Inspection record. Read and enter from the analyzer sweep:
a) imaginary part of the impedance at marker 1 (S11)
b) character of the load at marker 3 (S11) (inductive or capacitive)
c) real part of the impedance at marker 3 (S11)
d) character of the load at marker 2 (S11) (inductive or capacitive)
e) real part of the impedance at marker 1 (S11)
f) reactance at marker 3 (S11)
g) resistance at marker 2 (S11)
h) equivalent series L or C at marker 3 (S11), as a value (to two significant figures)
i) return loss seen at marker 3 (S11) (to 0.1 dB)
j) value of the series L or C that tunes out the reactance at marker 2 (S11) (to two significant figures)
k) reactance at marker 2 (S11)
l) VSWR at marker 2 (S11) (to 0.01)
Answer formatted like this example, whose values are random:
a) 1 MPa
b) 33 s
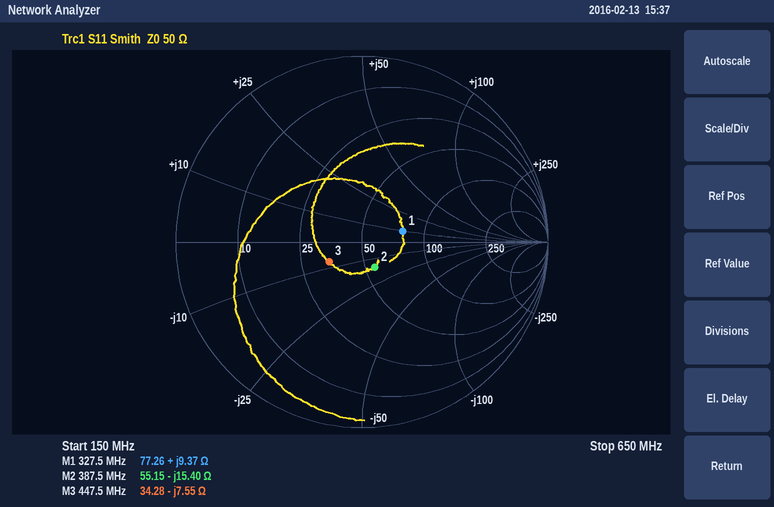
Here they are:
a) +9.37 Ω
b) capacitive
c) 34.28 Ω
d) capacitive
e) 77.26 Ω
f) -7.55 Ω
g) 55.15 Ω
h) 47 pF
i) 13.7 dB
j) 6.3 nH
k) -15.40 Ω
l) 1.36
